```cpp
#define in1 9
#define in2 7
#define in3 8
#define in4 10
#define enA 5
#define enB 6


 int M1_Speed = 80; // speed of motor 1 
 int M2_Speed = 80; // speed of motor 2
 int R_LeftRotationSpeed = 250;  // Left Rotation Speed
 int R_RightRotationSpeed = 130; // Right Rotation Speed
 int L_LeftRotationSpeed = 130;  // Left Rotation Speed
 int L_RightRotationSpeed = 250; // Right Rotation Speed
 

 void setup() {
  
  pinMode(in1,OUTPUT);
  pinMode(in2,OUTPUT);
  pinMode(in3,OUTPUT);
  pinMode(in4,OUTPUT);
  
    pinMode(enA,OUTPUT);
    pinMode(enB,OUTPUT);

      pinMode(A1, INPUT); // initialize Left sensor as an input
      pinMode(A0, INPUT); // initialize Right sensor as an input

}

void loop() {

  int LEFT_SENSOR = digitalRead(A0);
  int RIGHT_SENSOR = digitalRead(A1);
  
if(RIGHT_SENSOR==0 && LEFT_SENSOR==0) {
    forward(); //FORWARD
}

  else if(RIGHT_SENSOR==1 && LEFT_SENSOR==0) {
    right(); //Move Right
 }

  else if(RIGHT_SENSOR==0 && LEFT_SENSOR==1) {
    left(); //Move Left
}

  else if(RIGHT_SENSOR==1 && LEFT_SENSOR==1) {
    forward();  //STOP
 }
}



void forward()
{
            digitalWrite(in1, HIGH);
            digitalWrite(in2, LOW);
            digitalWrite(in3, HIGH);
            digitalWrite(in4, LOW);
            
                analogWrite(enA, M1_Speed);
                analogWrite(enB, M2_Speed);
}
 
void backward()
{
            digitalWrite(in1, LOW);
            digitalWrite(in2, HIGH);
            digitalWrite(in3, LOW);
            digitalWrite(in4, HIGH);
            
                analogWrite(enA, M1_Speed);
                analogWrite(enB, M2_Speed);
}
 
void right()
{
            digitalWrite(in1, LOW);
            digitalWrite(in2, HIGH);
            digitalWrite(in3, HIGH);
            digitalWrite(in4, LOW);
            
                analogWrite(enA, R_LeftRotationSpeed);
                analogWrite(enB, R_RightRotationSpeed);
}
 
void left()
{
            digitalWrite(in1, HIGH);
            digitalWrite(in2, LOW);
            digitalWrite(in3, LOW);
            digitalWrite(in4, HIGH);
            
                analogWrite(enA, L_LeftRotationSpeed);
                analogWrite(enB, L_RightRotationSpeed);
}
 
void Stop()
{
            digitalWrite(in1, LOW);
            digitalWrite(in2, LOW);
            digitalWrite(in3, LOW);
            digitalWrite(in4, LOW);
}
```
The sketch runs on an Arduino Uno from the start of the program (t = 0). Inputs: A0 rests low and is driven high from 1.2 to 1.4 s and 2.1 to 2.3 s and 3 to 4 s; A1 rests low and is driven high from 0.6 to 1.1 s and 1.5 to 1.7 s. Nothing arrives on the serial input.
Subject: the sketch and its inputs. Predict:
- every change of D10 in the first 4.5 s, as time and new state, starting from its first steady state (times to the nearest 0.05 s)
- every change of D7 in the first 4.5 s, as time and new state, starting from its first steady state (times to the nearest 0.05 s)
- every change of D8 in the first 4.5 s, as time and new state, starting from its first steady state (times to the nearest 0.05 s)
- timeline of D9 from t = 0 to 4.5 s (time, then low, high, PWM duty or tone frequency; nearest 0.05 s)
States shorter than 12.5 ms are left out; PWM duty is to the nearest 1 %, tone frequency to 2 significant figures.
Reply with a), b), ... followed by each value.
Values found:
a) 0 s low; 1.2 s high; 1.4 s low; 2.1 s high; 2.3 s low; 3 s high; 4 s low
b) 0 s low; 0.6 s high; 1.1 s low; 1.5 s high; 1.7 s low
c) 0 s high; 1.2 s low; 1.4 s high; 2.1 s low; 2.3 s high; 3 s low; 4 s high
d) 0 s high; 0.6 s low; 1.1 s high; 1.5 s low; 1.7 s high
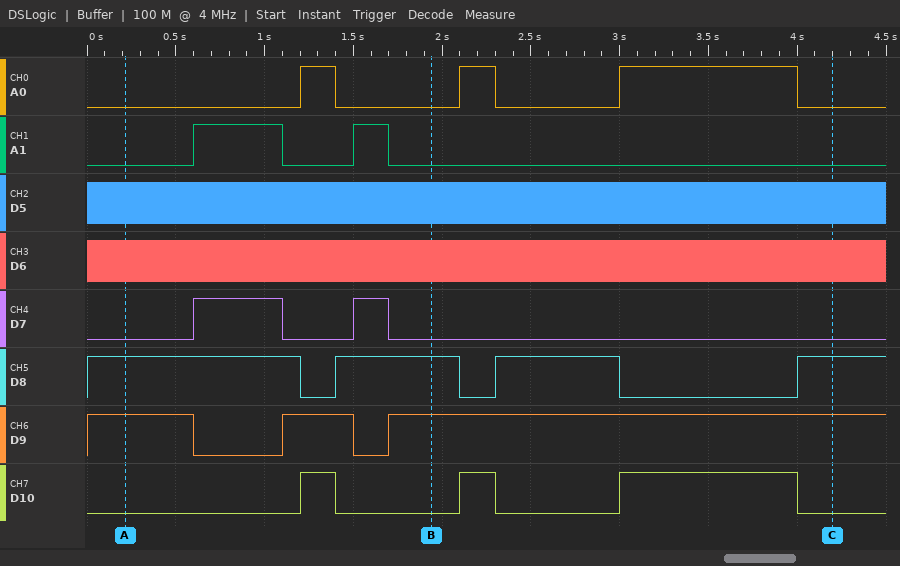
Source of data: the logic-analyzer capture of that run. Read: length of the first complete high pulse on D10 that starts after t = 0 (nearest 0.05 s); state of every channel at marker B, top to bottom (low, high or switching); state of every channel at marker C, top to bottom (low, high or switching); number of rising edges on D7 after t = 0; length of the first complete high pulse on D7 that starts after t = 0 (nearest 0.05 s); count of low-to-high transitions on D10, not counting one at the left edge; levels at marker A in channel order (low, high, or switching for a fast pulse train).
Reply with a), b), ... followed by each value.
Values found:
a) 0.20 s
b) A0 low, A1 low, D5 switching, D6 switching, D7 low, D8 high, D9 high, D10 low
c) A0 low, A1 low, D5 switching, D6 switching, D7 low, D8 high, D9 high, D10 low
d) 2
e) 0.50 s
f) 3
g) A0 low, A1 low, D5 switching, D6 switching, D7 low, D8 high, D9 high, D10 low
